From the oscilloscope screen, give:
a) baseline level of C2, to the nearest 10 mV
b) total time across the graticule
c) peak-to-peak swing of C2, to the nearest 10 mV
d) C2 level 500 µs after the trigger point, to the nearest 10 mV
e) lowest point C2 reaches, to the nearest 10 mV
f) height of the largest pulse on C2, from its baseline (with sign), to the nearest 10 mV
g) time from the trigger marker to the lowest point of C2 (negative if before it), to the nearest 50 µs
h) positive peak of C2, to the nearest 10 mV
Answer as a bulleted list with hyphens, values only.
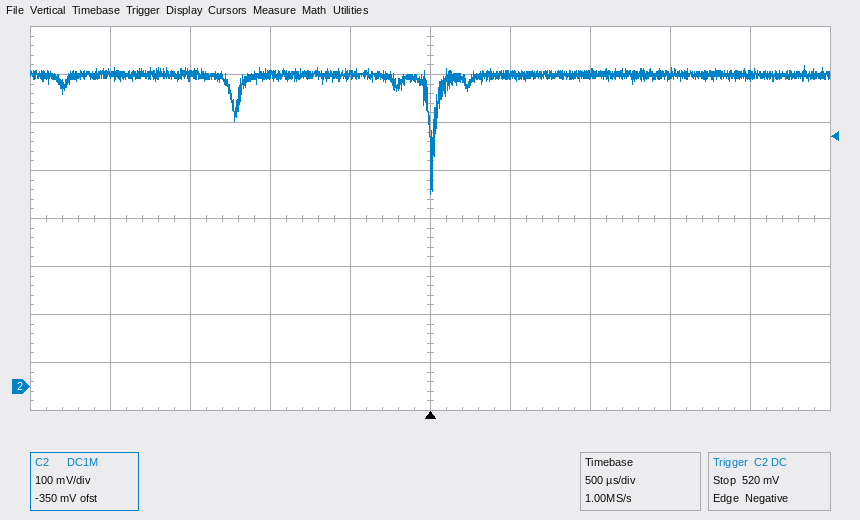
- 650 mV
- 5 ms
- 270 mV
- 650 mV
- 400 mV
- -250 mV
- 0 µs
- 670 mV
